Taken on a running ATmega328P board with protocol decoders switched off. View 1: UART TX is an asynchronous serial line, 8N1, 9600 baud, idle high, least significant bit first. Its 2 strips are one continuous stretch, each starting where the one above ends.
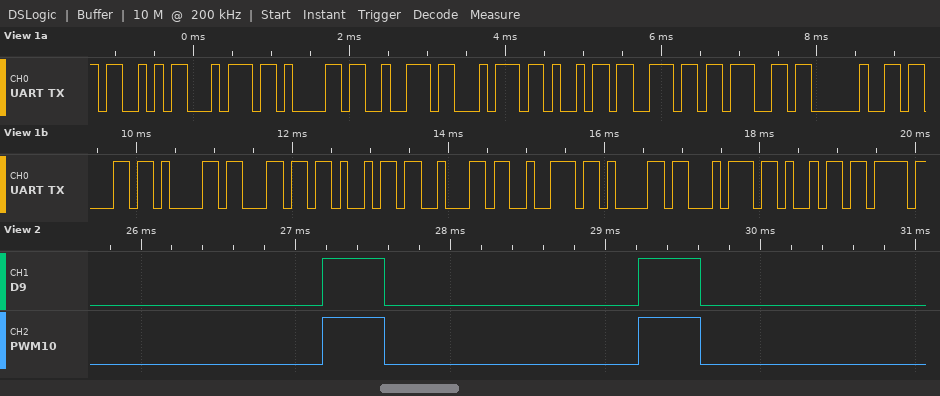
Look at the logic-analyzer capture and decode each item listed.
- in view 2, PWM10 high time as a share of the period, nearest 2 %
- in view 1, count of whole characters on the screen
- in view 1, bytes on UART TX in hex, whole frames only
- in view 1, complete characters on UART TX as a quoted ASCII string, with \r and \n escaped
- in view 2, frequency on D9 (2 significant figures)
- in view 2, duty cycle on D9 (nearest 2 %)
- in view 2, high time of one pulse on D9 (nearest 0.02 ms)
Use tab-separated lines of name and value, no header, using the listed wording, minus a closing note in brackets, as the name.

in view 2, PWM10 high time as a share of the period, nearest 2 %	20 %
in view 1, count of whole characters on the screen	18
in view 1, bytes on UART TX in hex, whole frames only	0x53 0x74 0x61 0x72 0x74 0x69 0x6E 0x67 0x20 0x63 0x61 0x6C 0x69 0x62 0x72 0x61 0x74 0x69
in view 1, complete characters on UART TX as a quoted ASCII string, with \r and \n escaped	"Starting calibrati"
in view 2, frequency on D9	490 Hz
in view 2, duty cycle on D9	20 %
in view 2, high time of one pulse on D9	0.40 ms
